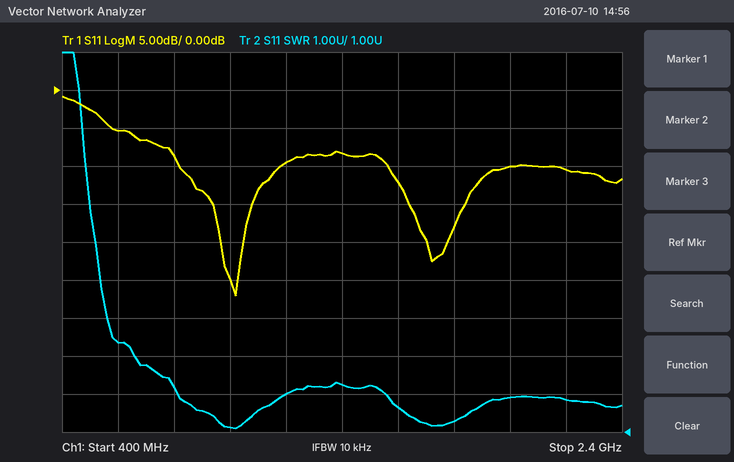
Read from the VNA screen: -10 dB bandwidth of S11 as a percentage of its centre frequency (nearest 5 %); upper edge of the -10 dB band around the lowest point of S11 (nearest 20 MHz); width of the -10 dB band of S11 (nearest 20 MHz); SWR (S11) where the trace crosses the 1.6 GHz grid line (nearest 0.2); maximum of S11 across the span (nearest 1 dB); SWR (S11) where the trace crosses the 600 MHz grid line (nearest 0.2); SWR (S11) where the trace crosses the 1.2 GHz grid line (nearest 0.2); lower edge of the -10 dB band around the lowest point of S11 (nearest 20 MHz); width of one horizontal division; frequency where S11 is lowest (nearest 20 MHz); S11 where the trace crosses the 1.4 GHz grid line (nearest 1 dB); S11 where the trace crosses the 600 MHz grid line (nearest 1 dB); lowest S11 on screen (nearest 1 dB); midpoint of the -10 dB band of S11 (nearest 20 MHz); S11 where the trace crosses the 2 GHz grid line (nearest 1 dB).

35 %
1.18 GHz
360 MHz
1.6
-1 dB
3.4
2.0
820 MHz
200 MHz
1.02 GHz
-8 dB
-5 dB
-27 dB
1.00 GHz
-10 dB
